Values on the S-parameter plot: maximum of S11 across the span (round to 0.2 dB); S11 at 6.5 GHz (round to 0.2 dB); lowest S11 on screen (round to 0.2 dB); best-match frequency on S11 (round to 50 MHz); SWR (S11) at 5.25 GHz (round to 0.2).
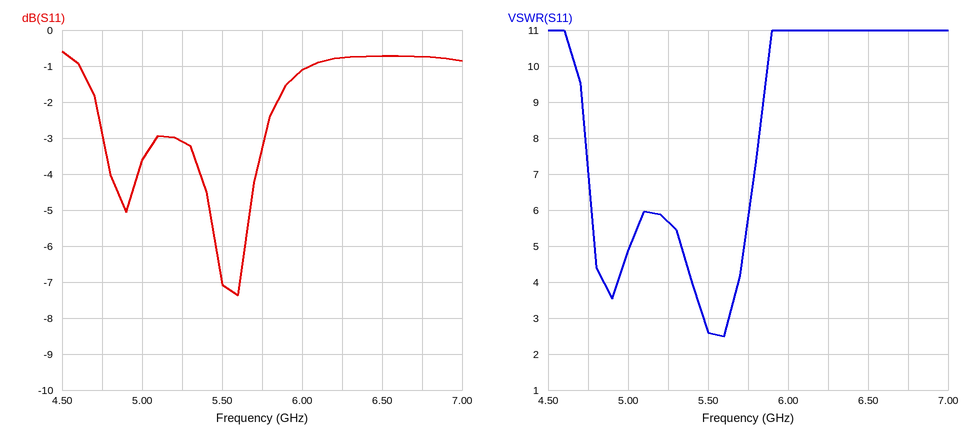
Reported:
-0.6 dB
-0.8 dB
-7.4 dB
5.60 GHz
5.6
